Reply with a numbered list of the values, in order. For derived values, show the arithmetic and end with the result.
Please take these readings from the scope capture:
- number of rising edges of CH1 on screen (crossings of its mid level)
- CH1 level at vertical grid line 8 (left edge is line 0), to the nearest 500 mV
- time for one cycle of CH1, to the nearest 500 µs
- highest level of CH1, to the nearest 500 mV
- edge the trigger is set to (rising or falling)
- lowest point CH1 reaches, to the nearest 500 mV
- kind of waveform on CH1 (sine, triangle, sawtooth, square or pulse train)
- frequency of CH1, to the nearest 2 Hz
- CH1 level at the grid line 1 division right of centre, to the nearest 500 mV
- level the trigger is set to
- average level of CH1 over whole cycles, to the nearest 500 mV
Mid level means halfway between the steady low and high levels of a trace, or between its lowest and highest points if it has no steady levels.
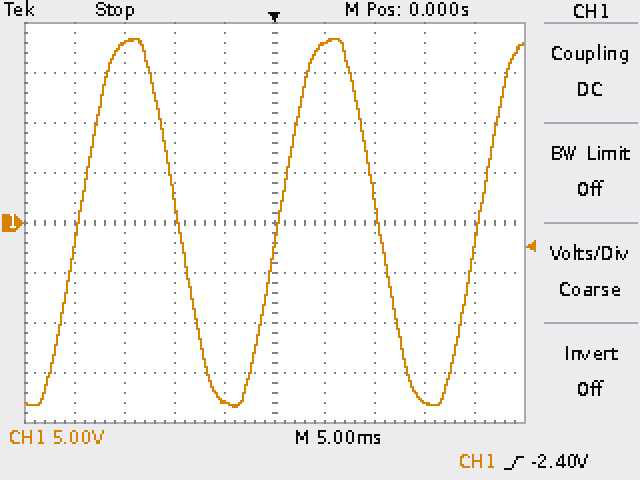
1. 3
2. -18.0 V
3. 20.0 ms
4. 18.5 V
5. rising
6. -18.5 V
7. sine
8. 1 / 20.0 ms ≈ 50 Hz
9. 18.0 V
10. -2.40 V
11. (18.5 V + (-18.5 V)) / 2 ≈ 0.0 V
